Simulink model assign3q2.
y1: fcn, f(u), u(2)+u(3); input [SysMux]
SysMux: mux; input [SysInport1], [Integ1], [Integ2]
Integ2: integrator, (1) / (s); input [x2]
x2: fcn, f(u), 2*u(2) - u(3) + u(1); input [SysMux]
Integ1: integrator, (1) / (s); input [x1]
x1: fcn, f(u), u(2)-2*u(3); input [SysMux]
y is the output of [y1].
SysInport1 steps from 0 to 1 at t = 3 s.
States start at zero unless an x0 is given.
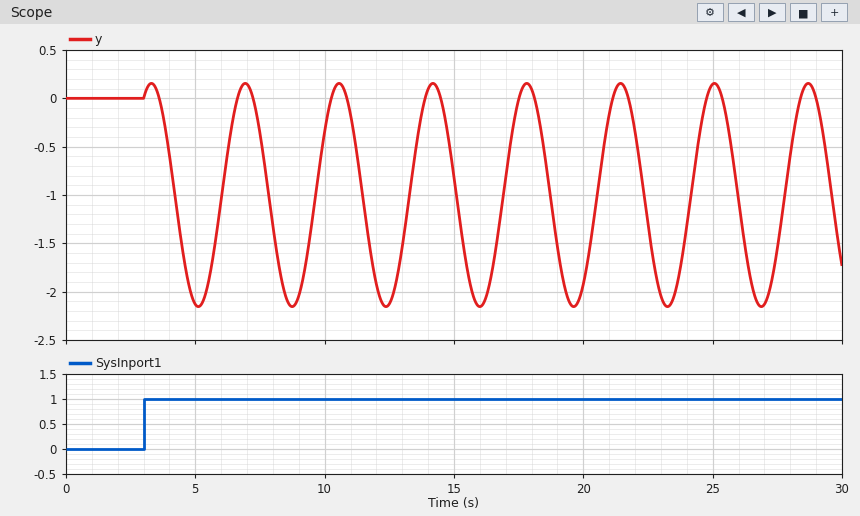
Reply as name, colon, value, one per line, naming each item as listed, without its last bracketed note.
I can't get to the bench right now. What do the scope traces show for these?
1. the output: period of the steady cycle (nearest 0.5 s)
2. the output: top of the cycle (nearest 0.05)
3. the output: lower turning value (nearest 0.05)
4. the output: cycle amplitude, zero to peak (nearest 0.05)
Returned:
the output: period of the steady cycle: 3.5 s
the output: top of the cycle: 0.15
the output: lower turning value: -2.15
the output: cycle amplitude, zero to peak: 1.15
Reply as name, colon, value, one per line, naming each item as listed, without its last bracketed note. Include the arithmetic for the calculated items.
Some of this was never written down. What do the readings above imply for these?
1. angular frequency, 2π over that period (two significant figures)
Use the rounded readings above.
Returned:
angular frequency, 2π over that period: 2π / 3.5 = 1.8 rad/s
